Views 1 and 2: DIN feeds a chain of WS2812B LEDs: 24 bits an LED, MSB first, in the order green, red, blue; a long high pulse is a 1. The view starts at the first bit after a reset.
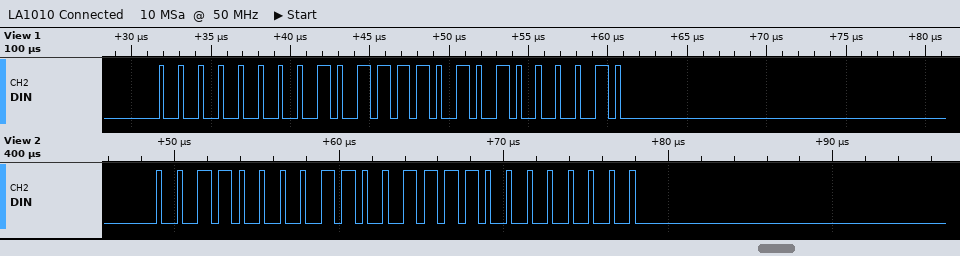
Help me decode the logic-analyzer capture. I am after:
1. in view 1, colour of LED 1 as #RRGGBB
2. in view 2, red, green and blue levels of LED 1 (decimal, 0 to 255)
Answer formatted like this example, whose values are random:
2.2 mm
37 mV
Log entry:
#BD0042
207, 48, 0
